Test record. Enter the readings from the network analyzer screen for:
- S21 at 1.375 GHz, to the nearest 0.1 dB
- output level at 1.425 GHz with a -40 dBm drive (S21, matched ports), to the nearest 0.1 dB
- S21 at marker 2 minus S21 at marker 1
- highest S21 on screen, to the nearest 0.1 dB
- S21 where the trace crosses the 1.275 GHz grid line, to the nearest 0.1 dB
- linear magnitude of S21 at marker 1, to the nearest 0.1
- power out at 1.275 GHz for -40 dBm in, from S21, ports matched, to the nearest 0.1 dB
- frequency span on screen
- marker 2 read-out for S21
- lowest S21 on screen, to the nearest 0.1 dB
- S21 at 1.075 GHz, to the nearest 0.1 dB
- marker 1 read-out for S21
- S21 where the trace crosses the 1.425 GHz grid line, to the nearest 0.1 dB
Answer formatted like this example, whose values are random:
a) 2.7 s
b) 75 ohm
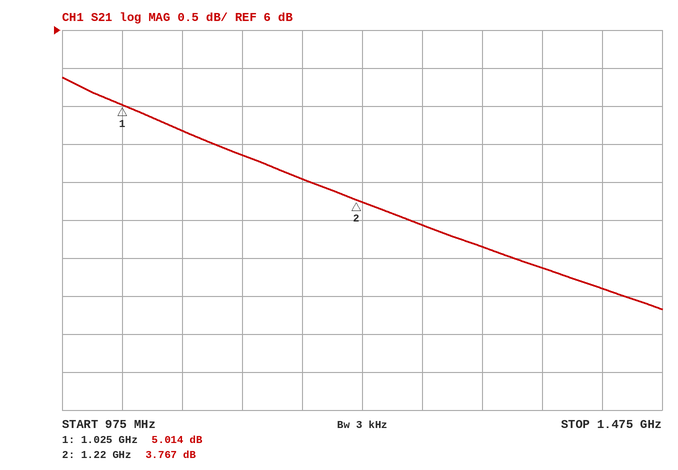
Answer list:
a) 2.9 dB
b) -37.4 dBm
c) -1.247 dB
d) 5.4 dB
e) 3.4 dB
f) 1.8
g) -36.6 dBm
h) 500 MHz
i) 3.767 dB
j) 2.3 dB
k) 4.7 dB
l) 5.014 dB
m) 2.6 dB
